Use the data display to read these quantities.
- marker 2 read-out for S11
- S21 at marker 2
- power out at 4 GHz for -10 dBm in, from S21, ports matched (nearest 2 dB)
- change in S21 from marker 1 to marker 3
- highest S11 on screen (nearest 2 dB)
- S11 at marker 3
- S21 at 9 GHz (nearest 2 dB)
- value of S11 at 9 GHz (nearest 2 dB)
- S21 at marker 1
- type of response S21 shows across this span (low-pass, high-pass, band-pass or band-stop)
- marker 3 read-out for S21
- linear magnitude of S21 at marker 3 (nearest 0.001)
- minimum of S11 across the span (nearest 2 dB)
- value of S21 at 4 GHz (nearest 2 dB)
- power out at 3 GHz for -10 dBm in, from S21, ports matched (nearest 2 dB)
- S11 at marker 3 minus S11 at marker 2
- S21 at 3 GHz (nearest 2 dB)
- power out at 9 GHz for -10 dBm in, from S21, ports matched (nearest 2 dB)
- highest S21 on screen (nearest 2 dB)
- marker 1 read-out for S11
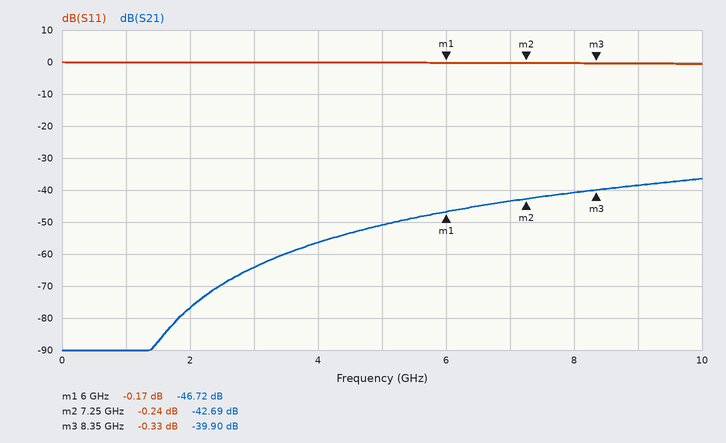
-0.24 dB
-42.69 dB
-66 dBm
6.82 dB
0 dB
-0.33 dB
-38 dB
0 dB
-46.72 dB
high-pass
-39.90 dB
0.010
0 dB
-56 dB
-74 dBm
-0.09 dB
-64 dB
-48 dBm
-36 dB
-0.17 dB
